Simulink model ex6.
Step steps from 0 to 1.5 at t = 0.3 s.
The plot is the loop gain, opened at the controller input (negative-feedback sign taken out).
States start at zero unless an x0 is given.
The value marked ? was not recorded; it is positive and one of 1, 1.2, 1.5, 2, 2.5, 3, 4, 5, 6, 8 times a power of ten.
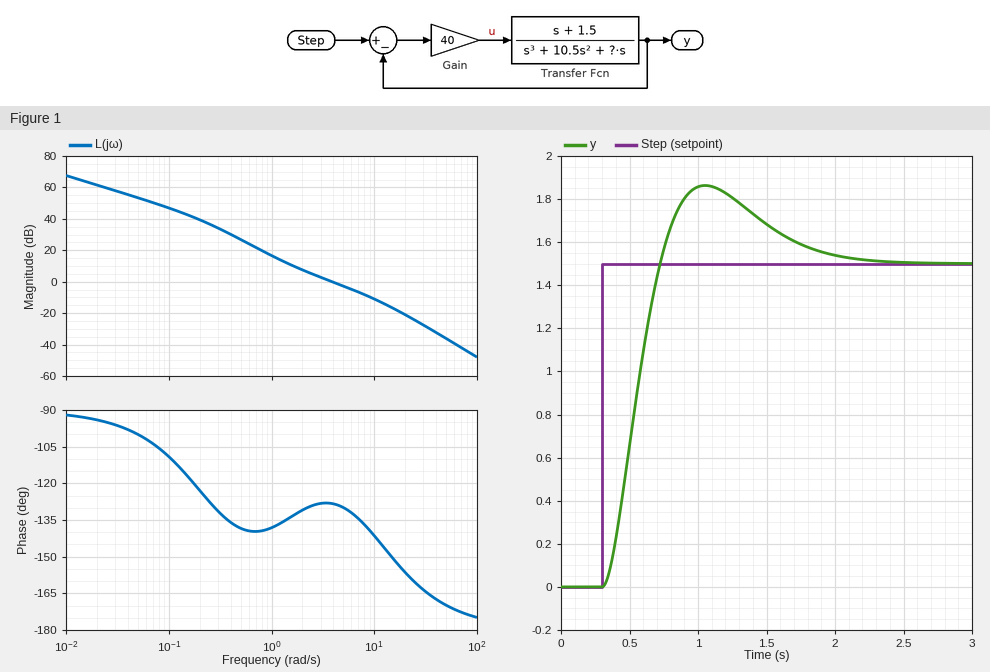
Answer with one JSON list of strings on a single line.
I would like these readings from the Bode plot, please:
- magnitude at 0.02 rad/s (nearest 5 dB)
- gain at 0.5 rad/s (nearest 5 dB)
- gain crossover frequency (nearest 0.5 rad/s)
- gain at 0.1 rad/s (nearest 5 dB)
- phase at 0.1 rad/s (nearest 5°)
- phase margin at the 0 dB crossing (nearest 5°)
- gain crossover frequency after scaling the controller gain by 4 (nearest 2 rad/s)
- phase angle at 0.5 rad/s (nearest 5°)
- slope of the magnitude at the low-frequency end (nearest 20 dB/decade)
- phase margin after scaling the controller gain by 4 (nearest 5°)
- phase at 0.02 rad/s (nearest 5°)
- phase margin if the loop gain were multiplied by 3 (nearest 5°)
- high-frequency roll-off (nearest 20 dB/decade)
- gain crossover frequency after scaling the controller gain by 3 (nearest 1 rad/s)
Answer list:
["60 dB", "25 dB", "4.0 rad/s", "45 dB", "-110°", "50°", "10 rad/s", "-140°", "-20 dB/decade", "35°", "-95°", "40°", "-40 dB/decade", "9 rad/s"]
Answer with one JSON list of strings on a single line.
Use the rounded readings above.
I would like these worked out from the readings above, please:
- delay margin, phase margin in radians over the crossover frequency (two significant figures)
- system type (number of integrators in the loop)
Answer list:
["0.22 s", "1"]
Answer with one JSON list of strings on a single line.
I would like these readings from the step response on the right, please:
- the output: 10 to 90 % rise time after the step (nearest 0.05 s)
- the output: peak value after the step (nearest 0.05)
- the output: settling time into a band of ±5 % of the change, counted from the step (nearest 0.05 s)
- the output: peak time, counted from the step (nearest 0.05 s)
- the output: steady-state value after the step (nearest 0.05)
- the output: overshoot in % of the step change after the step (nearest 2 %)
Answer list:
["0.30 s", "1.85", "1.50 s", "0.75 s", "1.50", "24 %"]
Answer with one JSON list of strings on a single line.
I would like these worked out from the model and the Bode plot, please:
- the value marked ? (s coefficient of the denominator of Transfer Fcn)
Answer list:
["2.5"]
